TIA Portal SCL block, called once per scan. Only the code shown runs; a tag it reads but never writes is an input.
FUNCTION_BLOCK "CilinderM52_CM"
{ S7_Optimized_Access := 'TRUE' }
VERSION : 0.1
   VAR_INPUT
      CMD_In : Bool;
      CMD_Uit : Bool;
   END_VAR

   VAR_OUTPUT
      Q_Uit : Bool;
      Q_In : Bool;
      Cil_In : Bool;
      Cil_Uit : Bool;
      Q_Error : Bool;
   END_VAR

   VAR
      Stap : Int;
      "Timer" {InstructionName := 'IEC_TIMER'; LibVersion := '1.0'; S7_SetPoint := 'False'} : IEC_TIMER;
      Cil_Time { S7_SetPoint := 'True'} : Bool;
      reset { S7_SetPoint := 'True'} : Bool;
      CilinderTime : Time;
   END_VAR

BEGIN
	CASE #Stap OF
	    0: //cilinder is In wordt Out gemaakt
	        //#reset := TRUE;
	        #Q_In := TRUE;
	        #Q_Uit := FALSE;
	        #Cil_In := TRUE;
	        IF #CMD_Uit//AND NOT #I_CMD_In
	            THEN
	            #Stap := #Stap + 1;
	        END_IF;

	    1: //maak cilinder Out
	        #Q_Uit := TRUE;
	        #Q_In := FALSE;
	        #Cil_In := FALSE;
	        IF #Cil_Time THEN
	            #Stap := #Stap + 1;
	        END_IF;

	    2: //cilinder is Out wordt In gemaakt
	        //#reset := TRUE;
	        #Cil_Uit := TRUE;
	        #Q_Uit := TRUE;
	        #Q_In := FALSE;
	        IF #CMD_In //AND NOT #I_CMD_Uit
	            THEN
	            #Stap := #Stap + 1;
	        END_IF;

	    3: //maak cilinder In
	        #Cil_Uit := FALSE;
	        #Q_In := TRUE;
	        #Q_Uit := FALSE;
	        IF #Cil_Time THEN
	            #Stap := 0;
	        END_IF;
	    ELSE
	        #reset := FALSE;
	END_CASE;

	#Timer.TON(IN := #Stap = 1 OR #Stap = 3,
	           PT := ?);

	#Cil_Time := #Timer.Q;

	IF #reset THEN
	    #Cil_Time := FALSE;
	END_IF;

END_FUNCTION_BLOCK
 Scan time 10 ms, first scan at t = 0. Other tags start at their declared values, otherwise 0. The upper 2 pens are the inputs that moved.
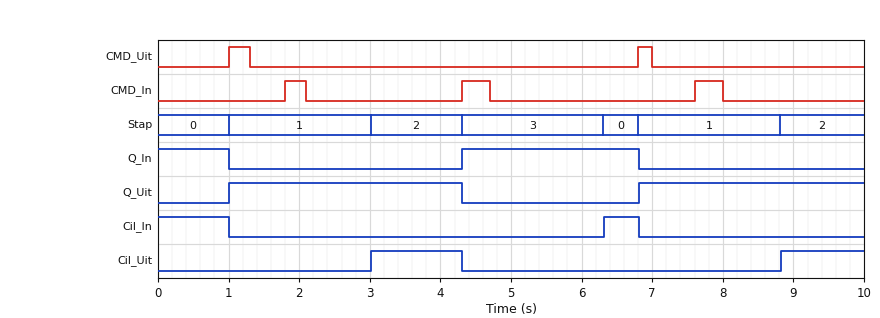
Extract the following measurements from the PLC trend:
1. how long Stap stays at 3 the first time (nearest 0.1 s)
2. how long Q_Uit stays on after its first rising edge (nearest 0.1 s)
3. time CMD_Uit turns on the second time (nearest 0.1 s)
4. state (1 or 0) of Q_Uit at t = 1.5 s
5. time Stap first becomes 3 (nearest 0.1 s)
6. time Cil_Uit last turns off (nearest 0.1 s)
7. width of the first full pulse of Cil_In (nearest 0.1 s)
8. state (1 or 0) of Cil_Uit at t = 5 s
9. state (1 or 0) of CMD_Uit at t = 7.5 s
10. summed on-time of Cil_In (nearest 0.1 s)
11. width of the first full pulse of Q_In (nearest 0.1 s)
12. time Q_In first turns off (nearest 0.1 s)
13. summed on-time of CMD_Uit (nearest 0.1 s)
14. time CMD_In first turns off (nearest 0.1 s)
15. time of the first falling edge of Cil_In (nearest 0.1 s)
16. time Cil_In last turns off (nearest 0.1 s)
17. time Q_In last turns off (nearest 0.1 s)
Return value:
2.0 s
3.3 s
6.8 s
1
4.3 s
4.3 s
0.5 s
0
0
1.5 s
2.5 s
1.0 s
0.5 s
2.1 s
1.0 s
6.8 s
6.8 s
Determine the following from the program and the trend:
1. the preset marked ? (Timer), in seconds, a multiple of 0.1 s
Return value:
2.0 s
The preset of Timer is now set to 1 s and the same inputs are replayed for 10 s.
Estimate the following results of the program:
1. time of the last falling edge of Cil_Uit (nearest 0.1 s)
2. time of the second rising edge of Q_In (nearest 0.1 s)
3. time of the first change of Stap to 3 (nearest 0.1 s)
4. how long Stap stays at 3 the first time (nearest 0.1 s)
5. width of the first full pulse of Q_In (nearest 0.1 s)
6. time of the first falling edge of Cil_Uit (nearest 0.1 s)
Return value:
7.8 s
7.8 s
2.0 s
1.0 s
4.8 s
2.0 s
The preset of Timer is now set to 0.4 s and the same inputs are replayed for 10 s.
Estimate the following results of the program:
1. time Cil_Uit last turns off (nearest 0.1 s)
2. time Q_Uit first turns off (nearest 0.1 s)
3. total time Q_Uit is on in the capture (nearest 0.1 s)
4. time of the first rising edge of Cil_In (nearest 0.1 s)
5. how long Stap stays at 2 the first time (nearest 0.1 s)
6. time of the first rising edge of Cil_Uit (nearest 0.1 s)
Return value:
7.6 s
1.8 s
1.6 s
2.2 s
0.4 s
1.4 s
